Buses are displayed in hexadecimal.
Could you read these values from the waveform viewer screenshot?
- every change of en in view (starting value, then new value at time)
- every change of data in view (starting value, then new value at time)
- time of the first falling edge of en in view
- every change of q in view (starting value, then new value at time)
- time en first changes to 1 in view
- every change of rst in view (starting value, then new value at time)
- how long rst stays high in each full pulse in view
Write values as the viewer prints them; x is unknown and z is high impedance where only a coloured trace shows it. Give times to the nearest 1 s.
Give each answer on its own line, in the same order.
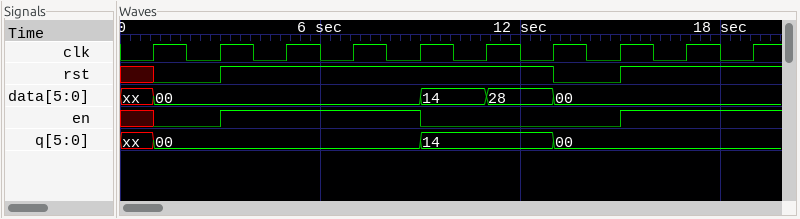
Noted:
x, 0 at 1 s, 1 at 3 s, 0 at 9 s, 1 at 15 s
xx, 00 at 1 s, 14 at 9 s, 28 at 11 s, 00 at 13 s
9 s
xx, 00 at 1 s, 14 at 9 s, 00 at 13 s
3 s
x, 0 at 1 s, 1 at 3 s, 0 at 13 s, 1 at 15 s
10 s
